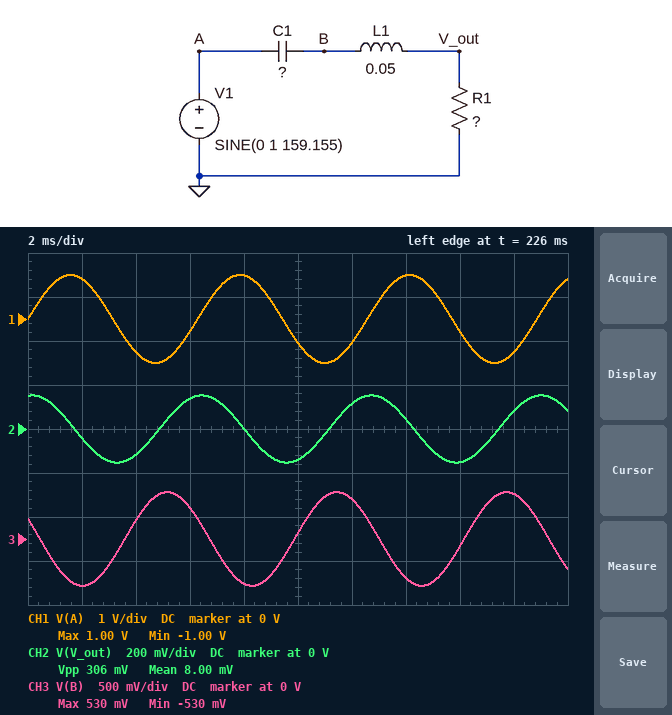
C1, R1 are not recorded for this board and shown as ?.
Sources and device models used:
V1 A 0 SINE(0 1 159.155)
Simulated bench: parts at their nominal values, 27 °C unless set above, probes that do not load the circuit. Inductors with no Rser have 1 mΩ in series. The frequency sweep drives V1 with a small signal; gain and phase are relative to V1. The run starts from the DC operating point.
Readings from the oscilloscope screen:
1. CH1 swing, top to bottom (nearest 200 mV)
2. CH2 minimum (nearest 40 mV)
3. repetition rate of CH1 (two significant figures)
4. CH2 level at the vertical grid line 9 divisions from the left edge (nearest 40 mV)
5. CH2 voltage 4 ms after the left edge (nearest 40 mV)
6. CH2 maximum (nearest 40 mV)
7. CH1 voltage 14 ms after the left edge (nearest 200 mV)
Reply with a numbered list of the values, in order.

1. 2.0 V
2. -160 mV
3. 160 Hz
4. 80 mV
5. -120 mV
6. 160 mV
7. 1.0 V
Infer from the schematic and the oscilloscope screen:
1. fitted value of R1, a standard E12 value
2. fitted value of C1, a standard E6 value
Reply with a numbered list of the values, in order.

1. 15 Ω
2. 6.8 µF
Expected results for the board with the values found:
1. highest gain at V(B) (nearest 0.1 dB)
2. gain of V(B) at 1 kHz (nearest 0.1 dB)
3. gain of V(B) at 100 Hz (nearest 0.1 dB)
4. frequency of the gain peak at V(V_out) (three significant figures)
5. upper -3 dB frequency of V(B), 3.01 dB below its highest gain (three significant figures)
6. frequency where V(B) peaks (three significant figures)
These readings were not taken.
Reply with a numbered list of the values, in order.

1. 15.3 dB
2. 0.7 dB
3. -15.3 dB
4. 273 Hz
5. 303 Hz
6. 275 Hz
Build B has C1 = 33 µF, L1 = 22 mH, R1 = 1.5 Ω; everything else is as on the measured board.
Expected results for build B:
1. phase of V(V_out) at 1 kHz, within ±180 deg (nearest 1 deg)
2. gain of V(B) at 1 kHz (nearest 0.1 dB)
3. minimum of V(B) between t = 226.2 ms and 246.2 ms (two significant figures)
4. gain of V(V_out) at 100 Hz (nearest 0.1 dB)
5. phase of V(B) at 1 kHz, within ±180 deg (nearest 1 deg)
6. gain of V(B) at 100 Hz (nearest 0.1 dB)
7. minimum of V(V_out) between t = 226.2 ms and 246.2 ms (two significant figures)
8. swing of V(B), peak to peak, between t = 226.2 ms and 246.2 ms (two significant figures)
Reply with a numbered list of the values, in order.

1. -89 deg
2. 0.3 dB
3. -2.6 V
4. -27.2 dB
5. 0 deg
6. -7.9 dB
7. -180 mV
8. 5.2 V
